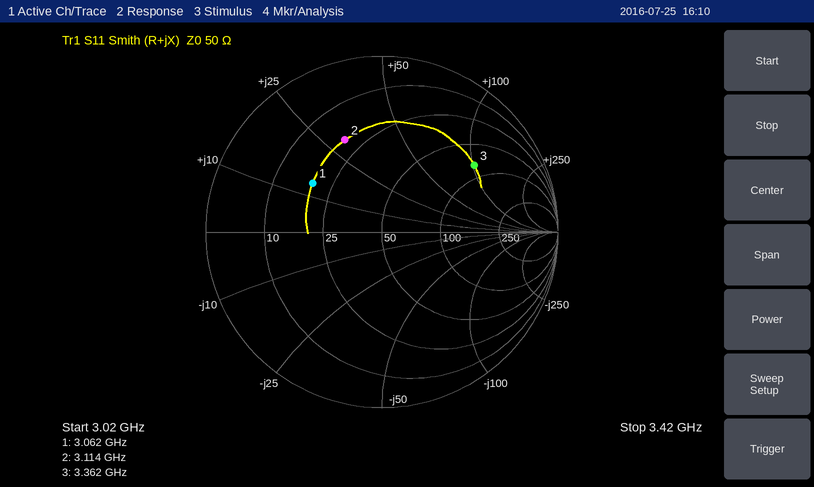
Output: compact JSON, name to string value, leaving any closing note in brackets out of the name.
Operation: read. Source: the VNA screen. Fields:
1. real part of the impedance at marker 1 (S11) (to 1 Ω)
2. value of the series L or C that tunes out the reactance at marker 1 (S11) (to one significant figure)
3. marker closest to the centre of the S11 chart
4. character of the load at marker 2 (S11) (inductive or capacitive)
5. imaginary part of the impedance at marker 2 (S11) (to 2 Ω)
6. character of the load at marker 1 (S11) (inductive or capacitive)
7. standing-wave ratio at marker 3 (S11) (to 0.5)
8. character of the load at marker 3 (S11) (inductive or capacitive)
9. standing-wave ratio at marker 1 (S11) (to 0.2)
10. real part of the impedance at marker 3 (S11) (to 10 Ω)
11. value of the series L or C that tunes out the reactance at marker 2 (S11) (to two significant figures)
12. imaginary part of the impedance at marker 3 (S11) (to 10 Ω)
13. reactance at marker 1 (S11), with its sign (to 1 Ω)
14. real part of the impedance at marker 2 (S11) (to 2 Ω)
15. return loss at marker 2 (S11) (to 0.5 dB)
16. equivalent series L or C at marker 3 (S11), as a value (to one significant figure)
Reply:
{"real part of the impedance at marker 1 (S11)": "19 Ω", "value of the series L or C that tunes out the reactance at marker 1 (S11)": "4 pF", "marker closest to the centre of the S11 chart": "marker 1", "character of the load at marker 2 (S11)": "inductive", "imaginary part of the impedance at marker 2 (S11)": "+30 Ω", "character of the load at marker 1 (S11)": "inductive", "standing-wave ratio at marker 3 (S11)": "4.5", "character of the load at marker 3 (S11)": "inductive", "standing-wave ratio at marker 1 (S11)": "2.8", "real part of the impedance at marker 3 (S11)": "80 Ω", "value of the series L or C that tunes out the reactance at marker 2 (S11)": "1.7 pF", "imaginary part of the impedance at marker 3 (S11)": "+100 Ω", "reactance at marker 1 (S11), with its sign": "+14 Ω", "real part of the impedance at marker 2 (S11)": "20 Ω", "return loss at marker 2 (S11)": "5.0 dB", "equivalent series L or C at marker 3 (S11), as a value": "5 nH"}
